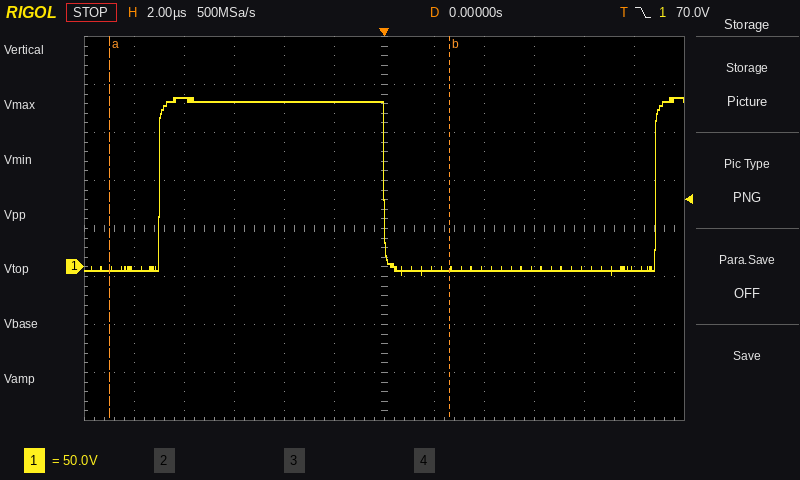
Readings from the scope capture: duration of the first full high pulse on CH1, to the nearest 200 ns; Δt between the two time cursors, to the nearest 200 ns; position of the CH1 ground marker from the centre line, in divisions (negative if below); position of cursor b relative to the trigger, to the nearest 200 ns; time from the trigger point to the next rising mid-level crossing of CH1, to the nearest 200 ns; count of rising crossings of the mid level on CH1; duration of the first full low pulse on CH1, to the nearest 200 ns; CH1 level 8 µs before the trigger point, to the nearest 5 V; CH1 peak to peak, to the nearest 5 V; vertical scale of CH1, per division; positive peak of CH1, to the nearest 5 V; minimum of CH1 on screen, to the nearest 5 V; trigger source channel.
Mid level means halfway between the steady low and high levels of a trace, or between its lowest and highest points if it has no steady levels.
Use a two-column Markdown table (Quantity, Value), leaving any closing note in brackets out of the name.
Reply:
| Quantity | Value |
|---|---|
| duration of the first full high pulse on CH1, to the nearest 200 ns | 9.0 µs |
| Δt between the two time cursors, to the nearest 200 ns | 13.6 µs |
| position of the CH1 ground marker from the centre line, in divisions | -0.8 div |
| position of cursor b relative to the trigger, to the nearest 200 ns | +2.6 µs |
| time from the trigger point to the next rising mid-level crossing of CH1, to the nearest 200 ns | 10.8 µs |
| count of rising crossings of the mid level on CH1 | 2 |
| duration of the first full low pulse on CH1, to the nearest 200 ns | 10.8 µs |
| CH1 level 8 µs before the trigger point, to the nearest 5 V | 175 V |
| CH1 peak to peak, to the nearest 5 V | 185 V |
| vertical scale of CH1, per division | 50 V |
| positive peak of CH1, to the nearest 5 V | 175 V |
| minimum of CH1 on screen, to the nearest 5 V | -10 V |
| trigger source channel | CH1 |
